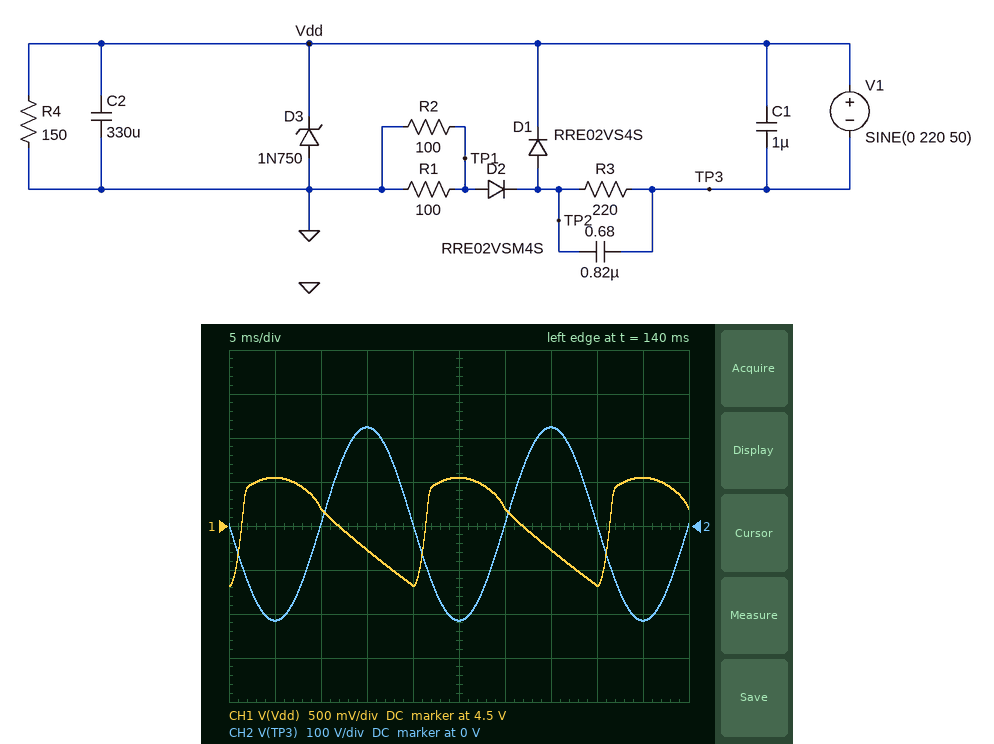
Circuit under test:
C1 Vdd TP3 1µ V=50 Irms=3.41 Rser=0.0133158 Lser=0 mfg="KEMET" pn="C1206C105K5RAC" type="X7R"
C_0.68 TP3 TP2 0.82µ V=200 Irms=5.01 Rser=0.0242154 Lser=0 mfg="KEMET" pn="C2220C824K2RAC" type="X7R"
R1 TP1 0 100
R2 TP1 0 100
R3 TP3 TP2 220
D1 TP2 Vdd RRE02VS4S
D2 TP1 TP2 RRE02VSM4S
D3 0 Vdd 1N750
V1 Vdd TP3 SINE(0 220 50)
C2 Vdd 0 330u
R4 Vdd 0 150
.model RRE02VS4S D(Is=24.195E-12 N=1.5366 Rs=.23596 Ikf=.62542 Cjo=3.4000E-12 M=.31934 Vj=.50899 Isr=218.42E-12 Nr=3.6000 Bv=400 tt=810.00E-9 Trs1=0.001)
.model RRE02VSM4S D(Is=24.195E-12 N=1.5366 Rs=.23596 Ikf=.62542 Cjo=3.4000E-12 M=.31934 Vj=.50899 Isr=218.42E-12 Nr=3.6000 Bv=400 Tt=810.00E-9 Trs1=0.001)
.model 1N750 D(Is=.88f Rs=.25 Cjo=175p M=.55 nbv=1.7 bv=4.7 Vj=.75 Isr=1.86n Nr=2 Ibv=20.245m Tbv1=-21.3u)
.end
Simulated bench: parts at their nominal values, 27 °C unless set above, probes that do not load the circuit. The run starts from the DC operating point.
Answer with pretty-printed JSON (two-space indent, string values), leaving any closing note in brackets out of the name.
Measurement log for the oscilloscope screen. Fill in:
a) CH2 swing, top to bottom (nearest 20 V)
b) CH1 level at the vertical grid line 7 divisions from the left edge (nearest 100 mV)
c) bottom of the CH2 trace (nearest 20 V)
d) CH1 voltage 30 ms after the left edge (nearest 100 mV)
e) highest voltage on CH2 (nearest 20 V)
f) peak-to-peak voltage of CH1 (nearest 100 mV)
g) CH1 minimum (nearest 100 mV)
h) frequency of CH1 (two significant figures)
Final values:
{
  "CH2 swing, top to bottom": "440 V",
  "CH1 level at the vertical grid line 7 divisions from the left edge": "4.2 V",
  "bottom of the CH2 trace": "-220 V",
  "CH1 voltage 30 ms after the left edge": "4.7 V",
  "highest voltage on CH2": "220 V",
  "peak-to-peak voltage of CH1": "1.2 V",
  "CH1 minimum": "3.8 V",
  "frequency of CH1": "50 Hz"
}
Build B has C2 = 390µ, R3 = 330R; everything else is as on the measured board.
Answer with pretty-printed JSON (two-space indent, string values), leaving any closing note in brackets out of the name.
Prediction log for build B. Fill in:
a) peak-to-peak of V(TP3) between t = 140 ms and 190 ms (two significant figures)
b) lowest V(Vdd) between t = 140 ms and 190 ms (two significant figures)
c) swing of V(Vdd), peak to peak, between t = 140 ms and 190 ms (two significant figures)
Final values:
{
  "peak-to-peak of V(TP3) between t = 140 ms and 190 ms": "440 V",
  "lowest V(Vdd) between t = 140 ms and 190 ms": "3.9 V",
  "swing of V(Vdd), peak to peak, between t = 140 ms and 190 ms": "1.0 V"
}
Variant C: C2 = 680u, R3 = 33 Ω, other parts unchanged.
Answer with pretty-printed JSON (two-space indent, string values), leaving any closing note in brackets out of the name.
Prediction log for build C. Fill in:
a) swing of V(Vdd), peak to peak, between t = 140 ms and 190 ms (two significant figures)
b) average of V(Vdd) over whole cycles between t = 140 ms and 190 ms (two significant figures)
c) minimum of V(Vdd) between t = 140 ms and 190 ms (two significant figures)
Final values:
{
  "swing of V(Vdd), peak to peak, between t = 140 ms and 190 ms": "1.3 V",
  "average of V(Vdd) over whole cycles between t = 140 ms and 190 ms": "4.9 V",
  "minimum of V(Vdd) between t = 140 ms and 190 ms": "4.3 V"
}
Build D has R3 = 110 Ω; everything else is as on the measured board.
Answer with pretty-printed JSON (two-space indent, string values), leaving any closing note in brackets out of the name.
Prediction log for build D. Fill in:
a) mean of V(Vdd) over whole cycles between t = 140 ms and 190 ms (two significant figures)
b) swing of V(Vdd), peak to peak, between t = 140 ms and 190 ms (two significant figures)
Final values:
{
  "mean of V(Vdd) over whole cycles between t = 140 ms and 190 ms": "4.6 V",
  "swing of V(Vdd), peak to peak, between t = 140 ms and 190 ms": "1.4 V"
}
